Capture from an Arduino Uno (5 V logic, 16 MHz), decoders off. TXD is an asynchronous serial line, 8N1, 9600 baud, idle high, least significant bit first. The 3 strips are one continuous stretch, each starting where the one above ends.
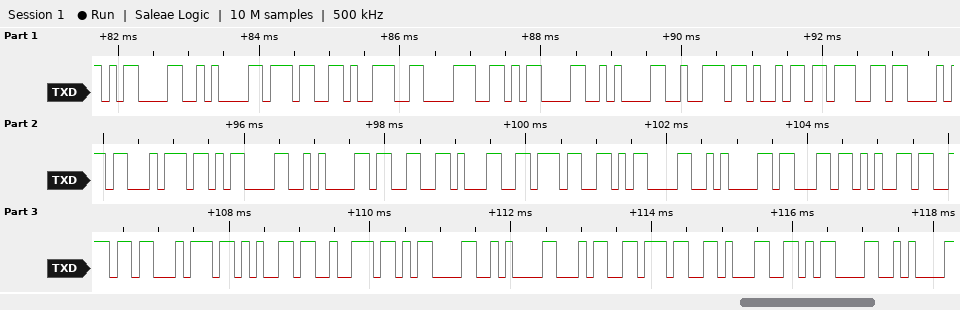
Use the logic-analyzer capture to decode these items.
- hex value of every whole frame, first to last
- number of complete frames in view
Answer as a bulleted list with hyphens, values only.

- 0D 0A 37 39 38 0D 0A 72 69 67 68 74 0D 0A 33 31 37 0D 0A 63 65 6E 74 65 72 0D 0A 34 37 31 0D 0A
- 32
